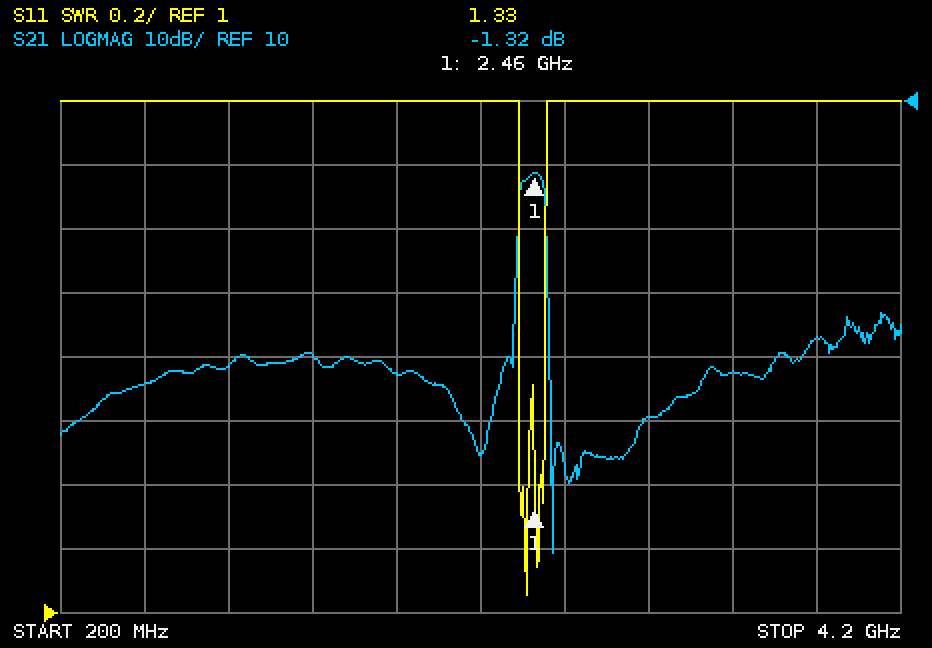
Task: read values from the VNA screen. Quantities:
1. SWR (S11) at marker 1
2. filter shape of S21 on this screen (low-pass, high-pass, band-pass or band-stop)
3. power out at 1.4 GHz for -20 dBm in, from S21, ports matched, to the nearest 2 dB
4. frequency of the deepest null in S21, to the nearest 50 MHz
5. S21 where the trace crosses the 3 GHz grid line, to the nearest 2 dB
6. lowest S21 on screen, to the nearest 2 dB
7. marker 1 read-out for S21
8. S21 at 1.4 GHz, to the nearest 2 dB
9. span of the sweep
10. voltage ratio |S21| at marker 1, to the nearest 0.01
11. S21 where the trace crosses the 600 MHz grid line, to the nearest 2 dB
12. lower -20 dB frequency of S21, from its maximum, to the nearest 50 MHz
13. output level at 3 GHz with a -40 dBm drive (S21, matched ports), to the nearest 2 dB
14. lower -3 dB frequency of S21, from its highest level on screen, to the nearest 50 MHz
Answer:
1.33
band-pass
-50 dBm
2.55 GHz
-40 dB
-60 dB
-1.32 dB
-30 dB
4 GHz
0.86
-34 dB
2.35 GHz
-80 dBm
2.40 GHz
